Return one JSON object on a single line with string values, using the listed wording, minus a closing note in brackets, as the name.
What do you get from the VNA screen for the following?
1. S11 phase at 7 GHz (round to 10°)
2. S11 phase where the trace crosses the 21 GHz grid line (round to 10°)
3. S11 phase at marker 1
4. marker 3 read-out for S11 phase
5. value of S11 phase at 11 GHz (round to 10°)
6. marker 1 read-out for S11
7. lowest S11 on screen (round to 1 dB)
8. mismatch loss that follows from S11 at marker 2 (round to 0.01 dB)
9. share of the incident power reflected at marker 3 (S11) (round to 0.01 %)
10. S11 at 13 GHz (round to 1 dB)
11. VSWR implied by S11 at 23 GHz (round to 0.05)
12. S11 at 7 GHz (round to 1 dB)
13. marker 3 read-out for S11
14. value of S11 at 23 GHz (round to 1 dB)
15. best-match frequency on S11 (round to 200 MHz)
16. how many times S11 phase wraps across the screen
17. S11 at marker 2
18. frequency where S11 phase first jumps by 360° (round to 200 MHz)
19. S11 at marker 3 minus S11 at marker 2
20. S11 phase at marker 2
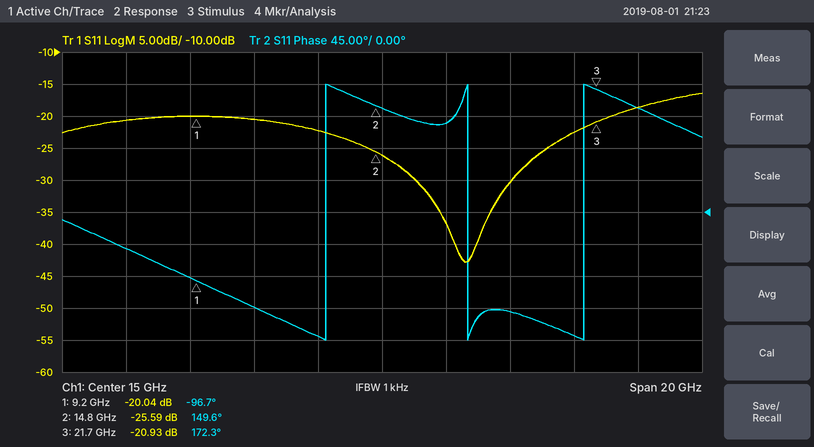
{"S11 phase at 7 GHz": "-50°", "S11 phase where the trace crosses the 21 GHz grid line": "-170°", "S11 phase at marker 1": "-96.7°", "marker 3 read-out for S11 phase": "172.3°", "value of S11 phase at 11 GHz": "-130°", "marker 1 read-out for S11": "-20.04 dB", "lowest S11 on screen": "-43 dB", "mismatch loss that follows from S11 at marker 2": "0.01 dB", "share of the incident power reflected at marker 3 (S11)": "0.81 %", "S11 at 13 GHz": "-22 dB", "VSWR implied by S11 at 23 GHz": "1.25", "S11 at 7 GHz": "-21 dB", "marker 3 read-out for S11": "-20.93 dB", "value of S11 at 23 GHz": "-19 dB", "best-match frequency on S11": "17.6 GHz", "how many times S11 phase wraps across the screen": "3", "S11 at marker 2": "-25.59 dB", "frequency where S11 phase first jumps by 360°": "13.2 GHz", "S11 at marker 3 minus S11 at marker 2": "4.66 dB", "S11 phase at marker 2": "149.6°"}
